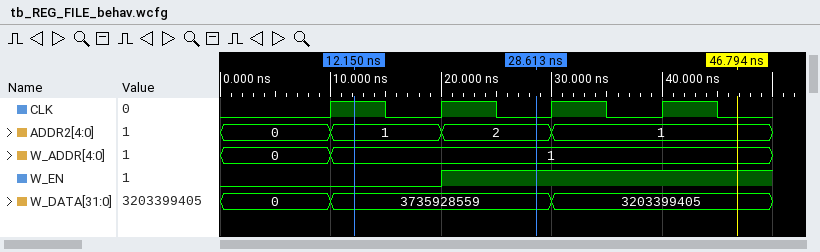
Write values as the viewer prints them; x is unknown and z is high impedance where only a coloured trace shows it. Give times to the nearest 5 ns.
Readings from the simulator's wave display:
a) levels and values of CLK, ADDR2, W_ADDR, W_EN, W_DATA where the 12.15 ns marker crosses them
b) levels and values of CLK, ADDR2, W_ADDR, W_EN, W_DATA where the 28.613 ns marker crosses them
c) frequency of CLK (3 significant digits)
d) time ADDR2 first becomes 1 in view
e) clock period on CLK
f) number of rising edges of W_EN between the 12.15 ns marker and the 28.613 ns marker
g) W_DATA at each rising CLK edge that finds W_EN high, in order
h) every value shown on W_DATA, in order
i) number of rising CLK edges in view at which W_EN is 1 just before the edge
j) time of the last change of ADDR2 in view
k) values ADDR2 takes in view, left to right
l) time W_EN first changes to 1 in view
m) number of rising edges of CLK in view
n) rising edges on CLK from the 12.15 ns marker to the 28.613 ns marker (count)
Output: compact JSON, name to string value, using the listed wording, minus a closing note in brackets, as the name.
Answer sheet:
{"levels and values of CLK, ADDR2, W_ADDR, W_EN, W_DATA where the 12.15 ns marker crosses them": "CLK=1, ADDR2=1, W_ADDR=1, W_EN=0, W_DATA=3735928559", "levels and values of CLK, ADDR2, W_ADDR, W_EN, W_DATA where the 28.613 ns marker crosses them": "CLK=0, ADDR2=2, W_ADDR=1, W_EN=1, W_DATA=3735928559", "frequency of CLK": "100 MHz", "time ADDR2 first becomes 1 in view": "10 ns", "clock period on CLK": "10 ns", "number of rising edges of W_EN between the 12.15 ns marker and the 28.613 ns marker": "1", "W_DATA at each rising CLK edge that finds W_EN high, in order": "3735928559, 3203399405", "every value shown on W_DATA, in order": "0, 3735928559, 3203399405", "number of rising CLK edges in view at which W_EN is 1 just before the edge": "2", "time of the last change of ADDR2 in view": "30 ns", "values ADDR2 takes in view, left to right": "0, 1, 2, 1", "time W_EN first changes to 1 in view": "20 ns", "number of rising edges of CLK in view": "4", "rising edges on CLK from the 12.15 ns marker to the 28.613 ns marker": "1"}
